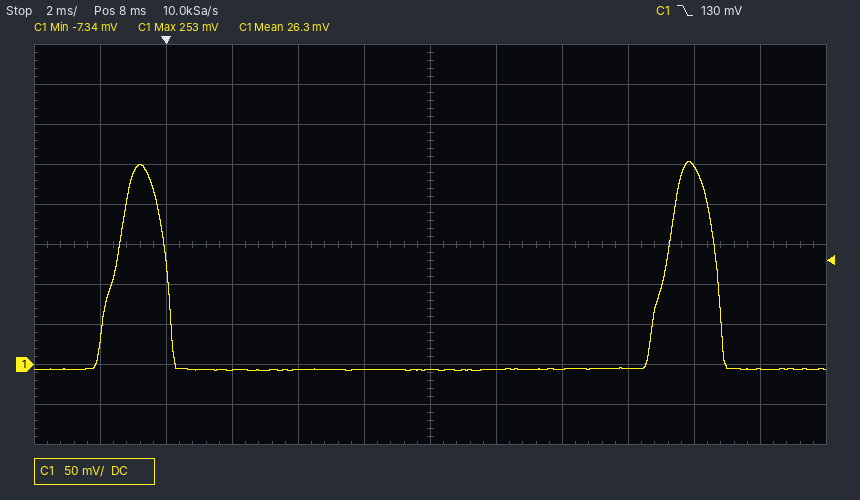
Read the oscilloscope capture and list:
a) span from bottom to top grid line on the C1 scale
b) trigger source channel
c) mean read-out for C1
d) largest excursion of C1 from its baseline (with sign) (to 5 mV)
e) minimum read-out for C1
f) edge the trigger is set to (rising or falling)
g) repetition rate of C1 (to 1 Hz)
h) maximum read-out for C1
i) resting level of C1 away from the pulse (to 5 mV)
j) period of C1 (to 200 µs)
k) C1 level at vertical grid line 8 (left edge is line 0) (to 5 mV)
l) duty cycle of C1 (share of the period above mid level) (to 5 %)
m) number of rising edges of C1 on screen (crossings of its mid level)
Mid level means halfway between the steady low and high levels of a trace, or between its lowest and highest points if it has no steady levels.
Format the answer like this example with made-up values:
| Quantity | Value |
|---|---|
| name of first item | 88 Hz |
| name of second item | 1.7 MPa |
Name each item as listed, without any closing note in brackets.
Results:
| Quantity | Value |
|---|---|
| span from bottom to top grid line on the C1 scale | 500 mV |
| trigger source channel | C1 |
| mean read-out for C1 | 26.3 mV |
| largest excursion of C1 from its baseline (with sign) | +260 mV |
| minimum read-out for C1 | -7.34 mV |
| edge the trigger is set to | falling |
| repetition rate of C1 | 60 Hz |
| maximum read-out for C1 | 253 mV |
| resting level of C1 away from the pulse | -5 mV |
| period of C1 | 16.6 ms |
| C1 level at vertical grid line 8 (left edge is line 0) | -5 mV |
| duty cycle of C1 (share of the period above mid level) | 10 % |
| number of rising edges of C1 on screen | 2 |
